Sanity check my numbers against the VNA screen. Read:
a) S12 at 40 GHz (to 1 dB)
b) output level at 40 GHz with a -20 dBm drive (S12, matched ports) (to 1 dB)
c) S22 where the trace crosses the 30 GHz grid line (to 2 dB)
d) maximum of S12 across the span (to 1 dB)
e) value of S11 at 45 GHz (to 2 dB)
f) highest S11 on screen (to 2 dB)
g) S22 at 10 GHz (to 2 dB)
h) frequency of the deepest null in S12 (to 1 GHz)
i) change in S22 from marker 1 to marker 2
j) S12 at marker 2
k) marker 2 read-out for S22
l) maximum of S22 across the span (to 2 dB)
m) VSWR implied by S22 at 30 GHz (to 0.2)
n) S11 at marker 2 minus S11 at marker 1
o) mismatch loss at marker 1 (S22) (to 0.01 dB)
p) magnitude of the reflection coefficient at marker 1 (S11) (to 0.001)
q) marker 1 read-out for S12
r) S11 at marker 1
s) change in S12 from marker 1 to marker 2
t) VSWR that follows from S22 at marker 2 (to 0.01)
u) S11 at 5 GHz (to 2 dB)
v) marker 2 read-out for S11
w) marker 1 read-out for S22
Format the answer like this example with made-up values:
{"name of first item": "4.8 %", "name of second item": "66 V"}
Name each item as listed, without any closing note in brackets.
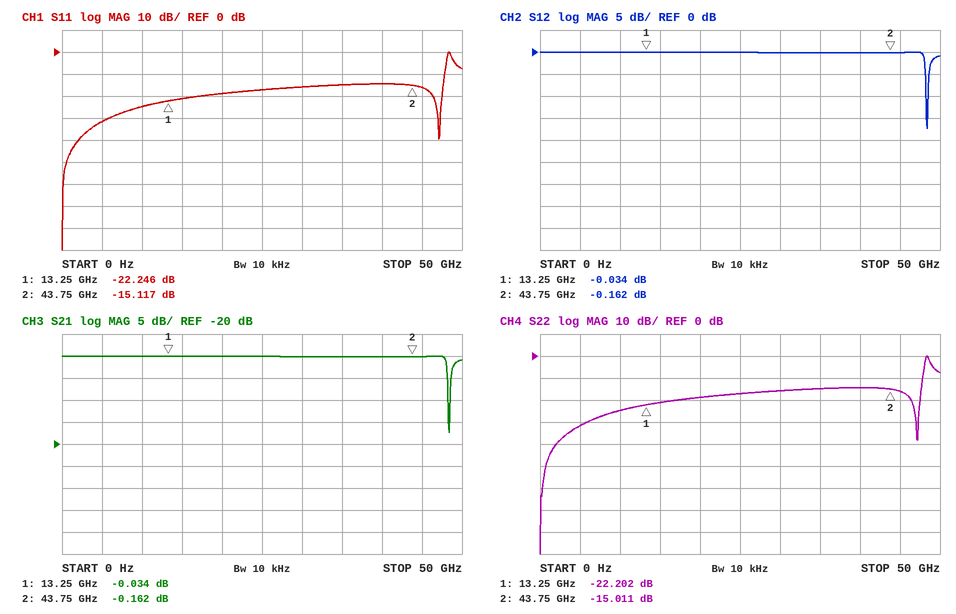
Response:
{"S12 at 40 GHz": "0 dB", "output level at 40 GHz with a -20 dBm drive (S12, matched ports)": "-20 dBm", "S22 where the trace crosses the 30 GHz grid line": "-16 dB", "maximum of S12 across the span": "0 dB", "value of S11 at 45 GHz": "-16 dB", "highest S11 on screen": "0 dB", "S22 at 10 GHz": "-24 dB", "frequency of the deepest null in S12": "48 GHz", "change in S22 from marker 1 to marker 2": "7.191 dB", "S12 at marker 2": "-0.162 dB", "marker 2 read-out for S22": "-15.011 dB", "maximum of S22 across the span": "0 dB", "VSWR implied by S22 at 30 GHz": "1.4", "S11 at marker 2 minus S11 at marker 1": "7.129 dB", "mismatch loss at marker 1 (S22)": "0.03 dB", "magnitude of the reflection coefficient at marker 1 (S11)": "0.077", "marker 1 read-out for S12": "-0.034 dB", "S11 at marker 1": "-22.246 dB", "change in S12 from marker 1 to marker 2": "-0.128 dB", "VSWR that follows from S22 at marker 2": "1.43", "S11 at 5 GHz": "-32 dB", "marker 2 read-out for S11": "-15.117 dB", "marker 1 read-out for S22": "-22.202 dB"}
